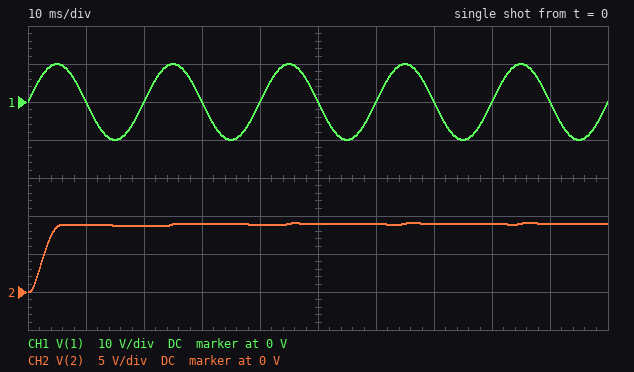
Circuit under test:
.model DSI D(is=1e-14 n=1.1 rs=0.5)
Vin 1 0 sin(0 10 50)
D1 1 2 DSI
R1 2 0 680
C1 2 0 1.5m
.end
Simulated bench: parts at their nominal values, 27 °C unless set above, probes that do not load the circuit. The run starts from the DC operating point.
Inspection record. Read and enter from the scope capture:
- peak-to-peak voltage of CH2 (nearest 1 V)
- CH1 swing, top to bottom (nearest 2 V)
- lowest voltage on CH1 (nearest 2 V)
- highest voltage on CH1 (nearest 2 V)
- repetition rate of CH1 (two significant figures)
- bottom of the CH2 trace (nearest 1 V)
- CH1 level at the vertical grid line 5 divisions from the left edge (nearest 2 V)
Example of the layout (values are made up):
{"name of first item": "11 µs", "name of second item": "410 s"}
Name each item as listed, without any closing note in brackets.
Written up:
{"peak-to-peak voltage of CH2": "9 V", "CH1 swing, top to bottom": "20 V", "lowest voltage on CH1": "-10 V", "highest voltage on CH1": "10 V", "repetition rate of CH1": "50 Hz", "bottom of the CH2 trace": "0 V", "CH1 level at the vertical grid line 5 divisions from the left edge": "0 V"}
